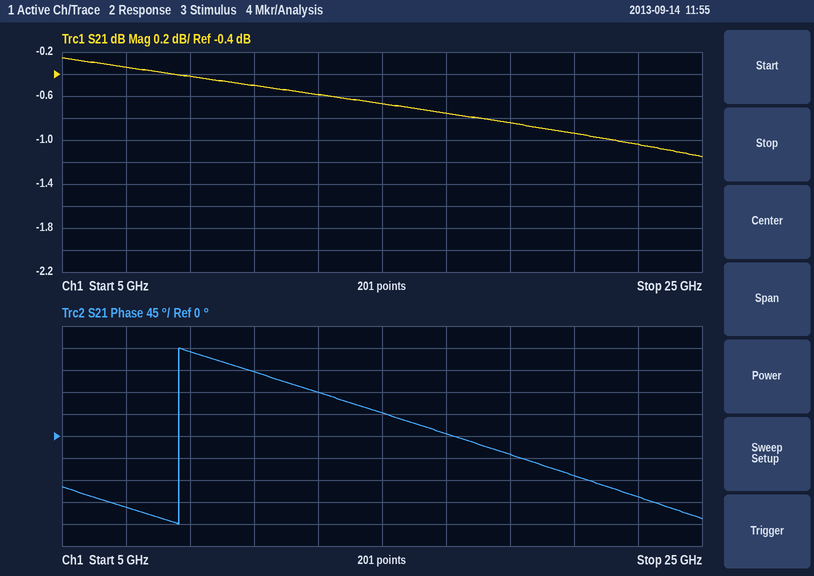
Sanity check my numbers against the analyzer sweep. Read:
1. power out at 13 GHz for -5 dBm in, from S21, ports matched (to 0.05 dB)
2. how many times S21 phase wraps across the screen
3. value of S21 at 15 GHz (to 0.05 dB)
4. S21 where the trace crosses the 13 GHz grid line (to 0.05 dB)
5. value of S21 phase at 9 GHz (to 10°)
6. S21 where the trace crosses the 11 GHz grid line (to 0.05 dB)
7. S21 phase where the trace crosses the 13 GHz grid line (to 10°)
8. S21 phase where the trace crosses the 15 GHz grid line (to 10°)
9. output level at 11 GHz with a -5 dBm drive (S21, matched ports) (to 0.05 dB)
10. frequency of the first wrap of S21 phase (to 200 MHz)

-5.60 dBm
1
-0.65 dB
-0.60 dB
170°
-0.50 dB
90°
50°
-5.50 dBm
8.6 GHz
